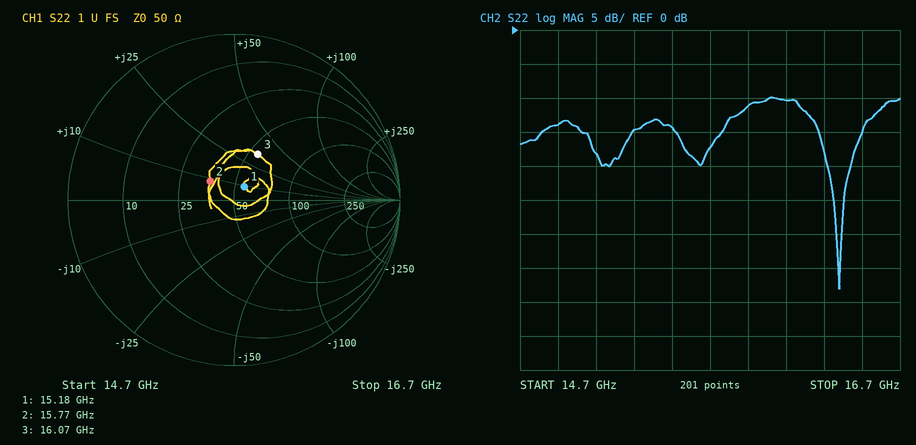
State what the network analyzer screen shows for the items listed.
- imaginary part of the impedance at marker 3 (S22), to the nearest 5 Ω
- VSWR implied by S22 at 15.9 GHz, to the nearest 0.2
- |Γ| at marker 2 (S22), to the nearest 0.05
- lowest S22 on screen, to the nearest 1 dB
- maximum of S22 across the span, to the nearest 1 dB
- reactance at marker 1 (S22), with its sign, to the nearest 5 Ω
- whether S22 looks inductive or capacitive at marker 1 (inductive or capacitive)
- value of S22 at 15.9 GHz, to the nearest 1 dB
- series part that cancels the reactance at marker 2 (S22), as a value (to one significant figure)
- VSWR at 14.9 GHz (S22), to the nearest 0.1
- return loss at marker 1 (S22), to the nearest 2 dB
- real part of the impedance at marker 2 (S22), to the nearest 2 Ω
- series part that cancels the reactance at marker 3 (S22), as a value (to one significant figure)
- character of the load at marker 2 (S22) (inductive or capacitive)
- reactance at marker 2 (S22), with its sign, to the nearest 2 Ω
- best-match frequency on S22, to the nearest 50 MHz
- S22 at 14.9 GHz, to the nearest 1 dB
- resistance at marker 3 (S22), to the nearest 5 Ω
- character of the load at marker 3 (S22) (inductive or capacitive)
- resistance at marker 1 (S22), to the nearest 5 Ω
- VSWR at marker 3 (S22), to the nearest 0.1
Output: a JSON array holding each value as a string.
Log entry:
["+35 Ω", "1.8", "0.20", "-38 dB", "-10 dB", "+10 Ω", "inductive", "-11 dB", "1 pF", "1.5", "20 dB", "36 Ω", "300 fF", "inductive", "+8 Ω", "16.40 GHz", "-14 dB", "55 Ω", "inductive", "55 Ω", "1.9"]
